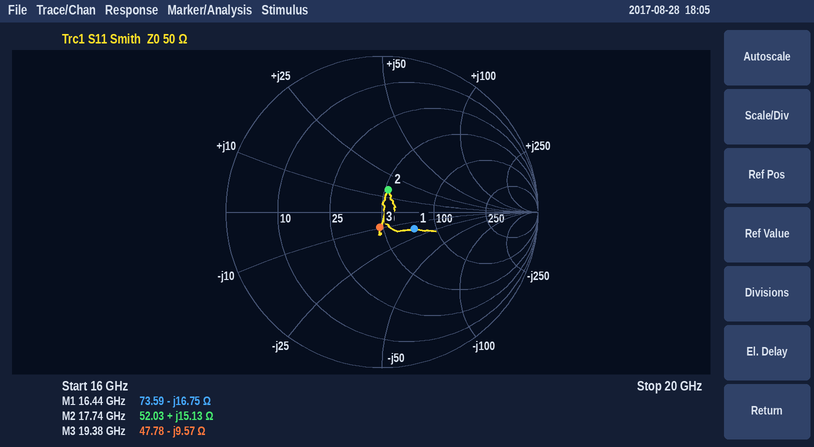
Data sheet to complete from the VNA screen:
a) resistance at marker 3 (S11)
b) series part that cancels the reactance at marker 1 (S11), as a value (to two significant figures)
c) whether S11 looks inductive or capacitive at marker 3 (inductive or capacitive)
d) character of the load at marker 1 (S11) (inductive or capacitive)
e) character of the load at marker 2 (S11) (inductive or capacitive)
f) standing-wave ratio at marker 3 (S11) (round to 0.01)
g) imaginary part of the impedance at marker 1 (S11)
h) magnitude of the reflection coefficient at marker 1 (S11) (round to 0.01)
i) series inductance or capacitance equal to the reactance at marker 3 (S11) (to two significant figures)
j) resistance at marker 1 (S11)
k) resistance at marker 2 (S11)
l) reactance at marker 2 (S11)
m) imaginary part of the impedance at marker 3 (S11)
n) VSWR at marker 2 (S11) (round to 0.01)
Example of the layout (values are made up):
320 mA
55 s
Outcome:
47.78 Ω
160 pH
capacitive
capacitive
inductive
1.22
-16.75 Ω
0.23
860 fF
73.59 Ω
52.03 Ω
+15.13 Ω
-9.57 Ω
1.35
